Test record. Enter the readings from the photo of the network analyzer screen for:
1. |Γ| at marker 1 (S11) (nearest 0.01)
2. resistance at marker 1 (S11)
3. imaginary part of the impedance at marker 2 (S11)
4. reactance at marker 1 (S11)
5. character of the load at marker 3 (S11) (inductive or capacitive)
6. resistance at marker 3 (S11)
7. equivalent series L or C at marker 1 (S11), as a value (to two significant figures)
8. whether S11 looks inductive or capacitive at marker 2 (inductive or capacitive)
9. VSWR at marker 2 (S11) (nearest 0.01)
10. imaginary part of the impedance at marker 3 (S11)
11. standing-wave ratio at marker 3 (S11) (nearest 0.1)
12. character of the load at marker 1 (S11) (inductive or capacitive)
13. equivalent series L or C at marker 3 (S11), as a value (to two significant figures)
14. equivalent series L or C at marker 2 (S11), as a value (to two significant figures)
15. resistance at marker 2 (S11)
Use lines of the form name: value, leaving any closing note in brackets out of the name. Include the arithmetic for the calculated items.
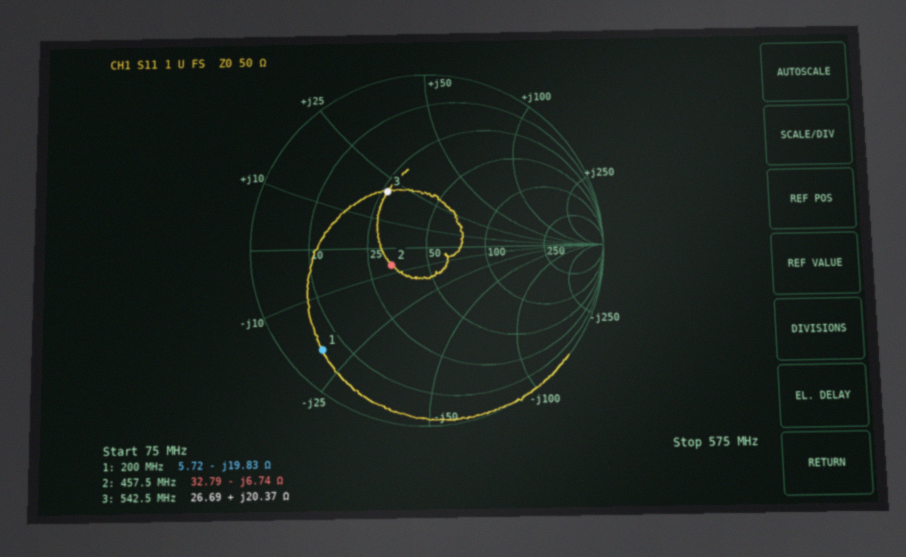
|Γ| at marker 1 (S11): 0.82
resistance at marker 1: 5.72 Ω
imaginary part of the impedance at marker 2: -6.74 Ω
reactance at marker 1: -19.83 Ω
character of the load at marker 3 (S11): inductive
resistance at marker 3: 26.69 Ω
equivalent series L or C at marker 1 (S11), as a value: C = 1/(2π × 200 MHz × 19.83 Ω) ≈ 40 pF
whether S11 looks inductive or capacitive at marker 2: capacitive
VSWR at marker 2 (S11): 1.57
imaginary part of the impedance at marker 3: +20.37 Ω
standing-wave ratio at marker 3 (S11): 2.3
character of the load at marker 1 (S11): capacitive
equivalent series L or C at marker 3 (S11), as a value: L = 20.37 Ω/(2π × 542.5 MHz) ≈ 6.0 nH
equivalent series L or C at marker 2 (S11), as a value: C = 1/(2π × 457.5 MHz × 6.74 Ω) ≈ 52 pF
resistance at marker 2: 32.79 Ω
